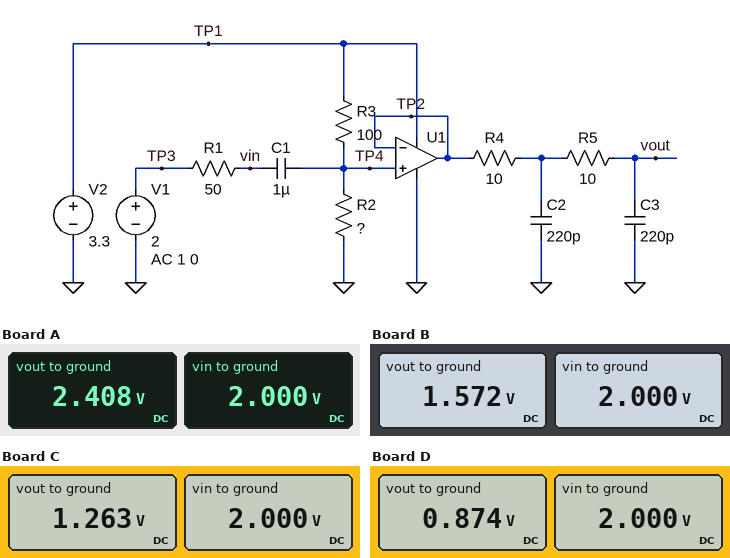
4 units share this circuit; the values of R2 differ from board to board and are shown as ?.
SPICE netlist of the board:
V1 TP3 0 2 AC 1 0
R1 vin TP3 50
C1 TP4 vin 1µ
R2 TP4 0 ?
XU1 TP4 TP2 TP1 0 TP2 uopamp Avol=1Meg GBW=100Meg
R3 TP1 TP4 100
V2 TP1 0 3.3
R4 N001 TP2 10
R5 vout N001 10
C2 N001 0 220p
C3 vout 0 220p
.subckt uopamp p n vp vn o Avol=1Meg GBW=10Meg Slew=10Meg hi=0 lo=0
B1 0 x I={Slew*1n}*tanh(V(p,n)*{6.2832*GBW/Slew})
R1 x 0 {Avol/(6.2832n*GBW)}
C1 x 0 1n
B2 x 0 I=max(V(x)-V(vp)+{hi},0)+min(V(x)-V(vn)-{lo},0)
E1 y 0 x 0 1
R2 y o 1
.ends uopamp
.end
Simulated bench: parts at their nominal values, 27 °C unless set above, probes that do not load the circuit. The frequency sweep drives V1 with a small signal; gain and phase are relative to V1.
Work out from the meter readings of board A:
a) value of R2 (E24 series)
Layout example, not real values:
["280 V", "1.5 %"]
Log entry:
["270 Ω"]
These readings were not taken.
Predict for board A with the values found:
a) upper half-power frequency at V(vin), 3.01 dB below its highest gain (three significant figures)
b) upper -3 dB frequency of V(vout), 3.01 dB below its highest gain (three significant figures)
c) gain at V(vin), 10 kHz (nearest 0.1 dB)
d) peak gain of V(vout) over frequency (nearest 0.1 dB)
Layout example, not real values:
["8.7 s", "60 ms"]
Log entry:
["2.38 kHz", "25.8 MHz", "-4.4 dB", "-4.5 dB"]
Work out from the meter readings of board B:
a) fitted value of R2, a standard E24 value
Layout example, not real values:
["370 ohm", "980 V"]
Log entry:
["91 Ω"]
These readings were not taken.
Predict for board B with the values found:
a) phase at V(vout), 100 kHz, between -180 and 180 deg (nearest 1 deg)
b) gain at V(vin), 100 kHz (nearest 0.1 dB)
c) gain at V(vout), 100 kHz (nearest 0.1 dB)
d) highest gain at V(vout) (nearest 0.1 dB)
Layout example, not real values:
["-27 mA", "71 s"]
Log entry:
["1 deg", "-6.2 dB", "-6.2 dB", "-6.2 dB"]
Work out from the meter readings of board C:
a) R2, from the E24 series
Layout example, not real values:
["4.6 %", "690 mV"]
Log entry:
["62 Ω"]
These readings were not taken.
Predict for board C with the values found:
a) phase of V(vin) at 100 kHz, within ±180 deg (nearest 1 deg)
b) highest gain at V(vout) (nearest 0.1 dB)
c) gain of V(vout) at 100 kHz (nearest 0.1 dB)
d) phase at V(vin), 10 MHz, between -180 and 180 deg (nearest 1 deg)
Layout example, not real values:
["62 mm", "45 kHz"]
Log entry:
["-1 deg", "-7.3 dB", "-7.3 dB", "0 deg"]
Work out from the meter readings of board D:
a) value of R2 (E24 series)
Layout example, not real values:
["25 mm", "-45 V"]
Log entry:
["36 Ω"]
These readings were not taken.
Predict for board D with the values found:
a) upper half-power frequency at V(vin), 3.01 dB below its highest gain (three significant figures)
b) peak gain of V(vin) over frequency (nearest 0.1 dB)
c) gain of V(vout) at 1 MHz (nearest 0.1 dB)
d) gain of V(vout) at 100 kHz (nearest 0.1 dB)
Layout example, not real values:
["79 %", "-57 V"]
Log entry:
["2.39 kHz", "0 dB", "-9.2 dB", "-9.2 dB"]
